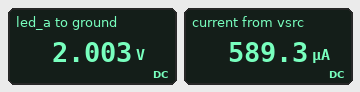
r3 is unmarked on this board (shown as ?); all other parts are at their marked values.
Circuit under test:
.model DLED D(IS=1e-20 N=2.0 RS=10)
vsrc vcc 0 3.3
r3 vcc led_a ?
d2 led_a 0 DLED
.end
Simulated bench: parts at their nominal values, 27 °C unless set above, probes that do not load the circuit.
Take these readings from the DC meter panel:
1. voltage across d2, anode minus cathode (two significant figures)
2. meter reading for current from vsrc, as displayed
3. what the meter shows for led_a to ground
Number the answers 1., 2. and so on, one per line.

1. 2.0 V
2. 589.3 µA
3. 2.003 V
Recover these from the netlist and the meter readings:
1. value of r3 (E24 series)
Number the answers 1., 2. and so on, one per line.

1. 2.2 kΩ
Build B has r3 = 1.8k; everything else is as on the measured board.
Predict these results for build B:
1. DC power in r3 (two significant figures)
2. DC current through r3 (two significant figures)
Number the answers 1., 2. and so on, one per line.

1. 920 µW
2. 710 µA
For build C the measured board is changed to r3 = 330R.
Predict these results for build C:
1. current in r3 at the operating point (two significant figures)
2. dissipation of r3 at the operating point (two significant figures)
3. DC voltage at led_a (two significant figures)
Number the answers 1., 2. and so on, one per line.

1. 3.6 mA
2. 4.2 mW
3. 2.1 V
